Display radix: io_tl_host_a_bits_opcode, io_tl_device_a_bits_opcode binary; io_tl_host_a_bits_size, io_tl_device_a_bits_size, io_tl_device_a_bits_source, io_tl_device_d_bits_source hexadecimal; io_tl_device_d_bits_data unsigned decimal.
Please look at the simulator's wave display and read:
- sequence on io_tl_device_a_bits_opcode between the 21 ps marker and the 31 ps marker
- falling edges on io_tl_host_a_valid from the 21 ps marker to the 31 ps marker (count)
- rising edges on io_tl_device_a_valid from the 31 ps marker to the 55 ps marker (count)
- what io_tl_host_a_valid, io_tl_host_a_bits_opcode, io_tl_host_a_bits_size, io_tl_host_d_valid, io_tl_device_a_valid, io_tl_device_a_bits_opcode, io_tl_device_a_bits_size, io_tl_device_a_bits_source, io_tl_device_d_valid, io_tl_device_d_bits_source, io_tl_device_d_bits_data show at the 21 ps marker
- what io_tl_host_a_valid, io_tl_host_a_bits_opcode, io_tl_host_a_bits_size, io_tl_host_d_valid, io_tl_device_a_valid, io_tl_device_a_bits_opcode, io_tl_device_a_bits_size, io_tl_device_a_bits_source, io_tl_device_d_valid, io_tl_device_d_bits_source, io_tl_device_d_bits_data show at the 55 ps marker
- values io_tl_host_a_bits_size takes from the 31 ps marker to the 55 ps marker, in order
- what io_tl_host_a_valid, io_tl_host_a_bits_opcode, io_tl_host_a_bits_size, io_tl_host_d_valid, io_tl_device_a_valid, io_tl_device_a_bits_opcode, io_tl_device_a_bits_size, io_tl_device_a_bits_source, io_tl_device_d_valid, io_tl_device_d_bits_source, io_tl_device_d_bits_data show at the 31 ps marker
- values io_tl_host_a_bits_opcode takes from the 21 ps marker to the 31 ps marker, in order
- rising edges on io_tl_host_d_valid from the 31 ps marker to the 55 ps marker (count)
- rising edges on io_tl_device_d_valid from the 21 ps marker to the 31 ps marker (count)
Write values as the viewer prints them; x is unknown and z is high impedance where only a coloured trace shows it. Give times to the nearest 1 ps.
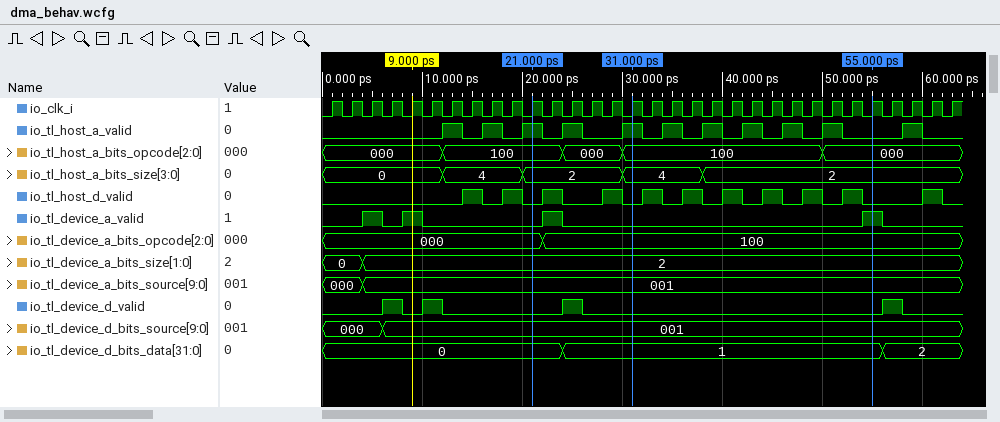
000, 100
2
1
io_tl_host_a_valid=1, io_tl_host_a_bits_opcode=100, io_tl_host_a_bits_size=2, io_tl_host_d_valid=0, io_tl_device_a_valid=0, io_tl_device_a_bits_opcode=000, io_tl_device_a_bits_size=2, io_tl_device_a_bits_source=001, io_tl_device_d_valid=0, io_tl_device_d_bits_source=001, io_tl_device_d_bits_data=0
io_tl_host_a_valid=0, io_tl_host_a_bits_opcode=000, io_tl_host_a_bits_size=2, io_tl_host_d_valid=0, io_tl_device_a_valid=1, io_tl_device_a_bits_opcode=100, io_tl_device_a_bits_size=2, io_tl_device_a_bits_source=001, io_tl_device_d_valid=0, io_tl_device_d_bits_source=001, io_tl_device_d_bits_data=1
4, 2
io_tl_host_a_valid=1, io_tl_host_a_bits_opcode=100, io_tl_host_a_bits_size=4, io_tl_host_d_valid=0, io_tl_device_a_valid=0, io_tl_device_a_bits_opcode=100, io_tl_device_a_bits_size=2, io_tl_device_a_bits_source=001, io_tl_device_d_valid=0, io_tl_device_d_bits_source=001, io_tl_device_d_bits_data=1
100, 000, 100
6
1
